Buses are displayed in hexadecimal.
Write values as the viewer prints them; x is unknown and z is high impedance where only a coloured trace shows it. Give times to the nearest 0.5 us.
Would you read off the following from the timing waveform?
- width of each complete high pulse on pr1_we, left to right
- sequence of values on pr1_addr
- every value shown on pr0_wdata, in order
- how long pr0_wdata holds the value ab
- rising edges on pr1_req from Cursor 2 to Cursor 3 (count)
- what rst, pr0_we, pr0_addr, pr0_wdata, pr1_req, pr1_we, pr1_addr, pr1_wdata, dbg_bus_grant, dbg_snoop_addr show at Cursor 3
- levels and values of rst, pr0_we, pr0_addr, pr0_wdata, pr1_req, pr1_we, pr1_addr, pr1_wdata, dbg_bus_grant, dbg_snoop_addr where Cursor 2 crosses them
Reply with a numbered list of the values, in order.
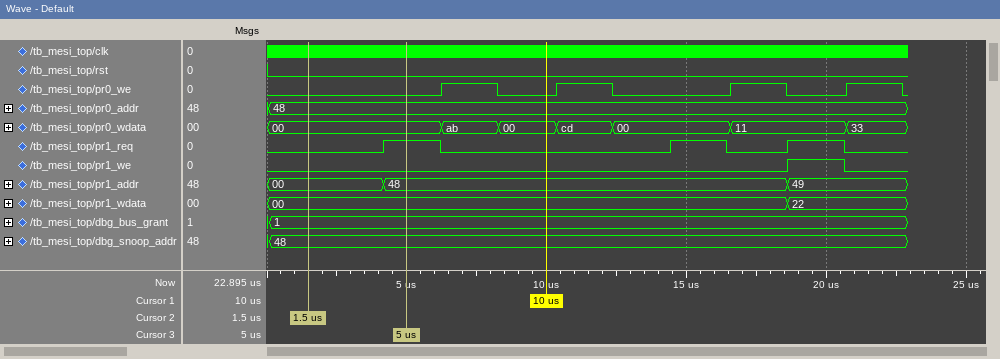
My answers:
1. 2 us
2. 00, 48, 49
3. 00, ab, 00, cd, 00, 11, 33
4. 2 us
5. 1
6. rst=0, pr0_we=0, pr0_addr=48, pr0_wdata=00, pr1_req=1, pr1_we=0, pr1_addr=48, pr1_wdata=00, dbg_bus_grant=1, dbg_snoop_addr=48
7. rst=0, pr0_we=0, pr0_addr=48, pr0_wdata=00, pr1_req=0, pr1_we=0, pr1_addr=00, pr1_wdata=00, dbg_bus_grant=1, dbg_snoop_addr=48
